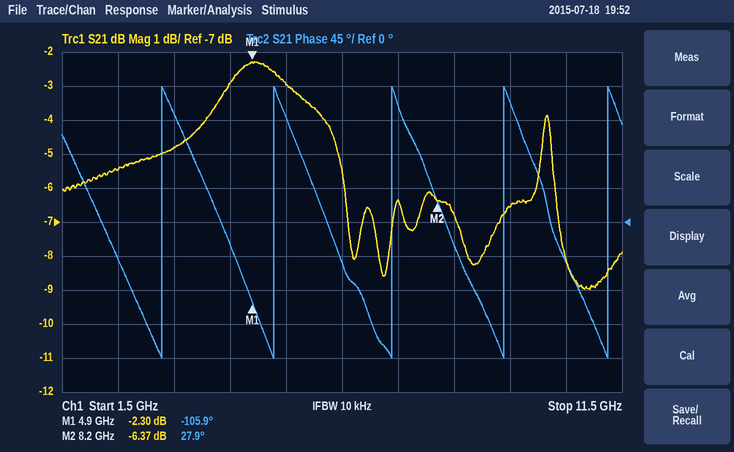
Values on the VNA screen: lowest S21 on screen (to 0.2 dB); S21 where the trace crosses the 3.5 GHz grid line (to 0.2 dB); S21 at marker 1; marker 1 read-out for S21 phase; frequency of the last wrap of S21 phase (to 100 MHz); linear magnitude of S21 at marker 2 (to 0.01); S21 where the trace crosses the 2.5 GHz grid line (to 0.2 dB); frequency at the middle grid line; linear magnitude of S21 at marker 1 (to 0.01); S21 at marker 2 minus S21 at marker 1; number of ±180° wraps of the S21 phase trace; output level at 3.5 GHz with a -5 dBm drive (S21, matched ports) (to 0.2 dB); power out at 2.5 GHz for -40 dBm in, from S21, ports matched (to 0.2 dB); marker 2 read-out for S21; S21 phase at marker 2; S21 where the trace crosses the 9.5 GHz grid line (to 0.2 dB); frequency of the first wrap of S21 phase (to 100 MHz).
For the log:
-9.0 dB
-4.8 dB
-2.30 dB
-105.9°
11.2 GHz
0.48
-5.4 dB
6.5 GHz
0.77
-4.07 dB
5
-9.8 dBm
-45.4 dBm
-6.37 dB
27.9°
-6.6 dB
3.3 GHz
